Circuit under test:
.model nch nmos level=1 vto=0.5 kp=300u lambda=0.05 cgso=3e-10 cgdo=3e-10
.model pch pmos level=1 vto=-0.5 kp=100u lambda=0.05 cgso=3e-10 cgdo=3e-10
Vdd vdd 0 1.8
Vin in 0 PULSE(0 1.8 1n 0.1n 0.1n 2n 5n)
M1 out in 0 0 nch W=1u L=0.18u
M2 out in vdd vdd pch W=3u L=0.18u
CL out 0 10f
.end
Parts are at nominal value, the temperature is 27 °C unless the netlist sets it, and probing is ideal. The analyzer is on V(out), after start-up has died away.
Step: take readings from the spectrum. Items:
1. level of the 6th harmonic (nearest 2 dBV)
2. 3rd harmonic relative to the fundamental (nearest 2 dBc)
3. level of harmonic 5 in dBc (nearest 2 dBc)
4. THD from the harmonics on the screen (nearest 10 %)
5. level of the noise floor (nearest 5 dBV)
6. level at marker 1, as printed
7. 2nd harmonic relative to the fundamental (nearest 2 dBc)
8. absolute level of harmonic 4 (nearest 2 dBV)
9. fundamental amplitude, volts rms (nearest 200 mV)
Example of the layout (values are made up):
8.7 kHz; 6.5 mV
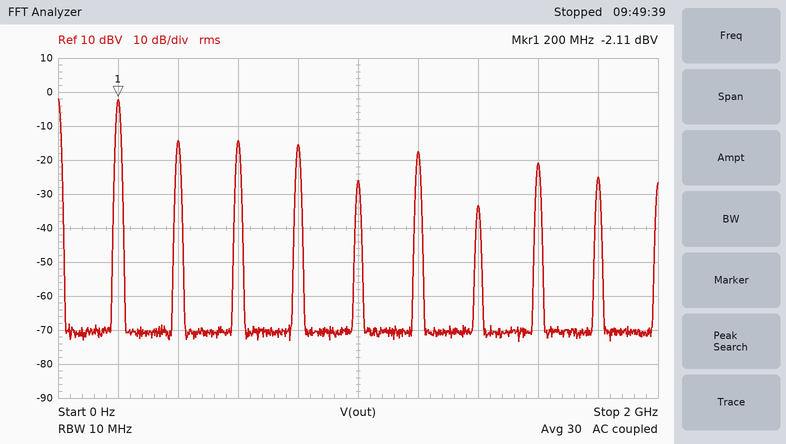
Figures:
-18 dBV; -12 dBc; -24 dBc; 50 %; -70 dBV; -2.11 dBV; -12 dBc; -16 dBV; 800 mV
